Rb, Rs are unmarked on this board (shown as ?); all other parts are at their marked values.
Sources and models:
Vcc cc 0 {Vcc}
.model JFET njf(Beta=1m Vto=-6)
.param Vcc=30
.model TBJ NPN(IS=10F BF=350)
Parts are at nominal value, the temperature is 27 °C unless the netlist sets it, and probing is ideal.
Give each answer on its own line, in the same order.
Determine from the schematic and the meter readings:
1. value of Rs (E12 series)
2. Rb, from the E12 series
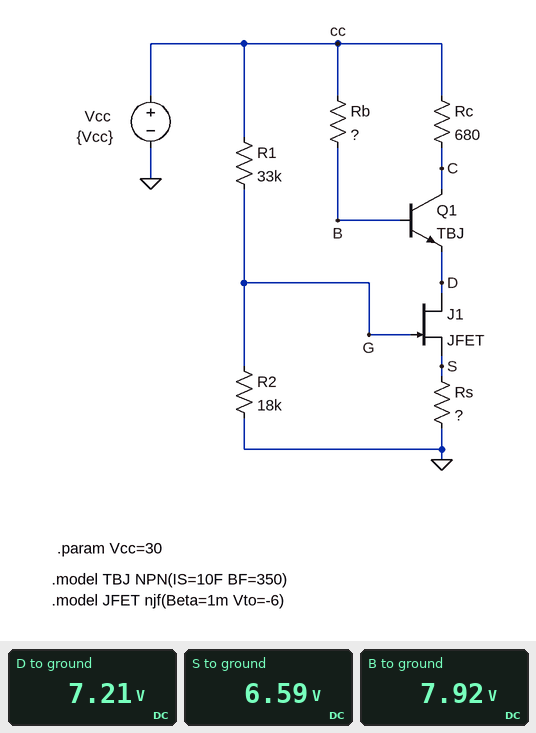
820 Ω
1 MΩ
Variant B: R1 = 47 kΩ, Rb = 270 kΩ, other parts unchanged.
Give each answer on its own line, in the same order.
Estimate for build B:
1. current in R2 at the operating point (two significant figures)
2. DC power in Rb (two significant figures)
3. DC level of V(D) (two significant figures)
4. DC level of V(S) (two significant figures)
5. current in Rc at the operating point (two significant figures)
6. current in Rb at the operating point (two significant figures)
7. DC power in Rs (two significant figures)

460 µA
370 µW
19 V
11 V
13 mA
37 µA
140 mW
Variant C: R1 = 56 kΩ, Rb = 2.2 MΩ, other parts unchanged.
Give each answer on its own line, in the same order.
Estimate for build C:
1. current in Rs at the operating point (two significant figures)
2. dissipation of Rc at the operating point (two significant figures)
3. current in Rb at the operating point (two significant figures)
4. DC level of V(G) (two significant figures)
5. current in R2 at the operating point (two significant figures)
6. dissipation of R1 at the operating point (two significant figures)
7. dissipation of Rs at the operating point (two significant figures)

4.3 mA
11 mW
12 µA
4.1 V
230 µA
12 mW
15 mW
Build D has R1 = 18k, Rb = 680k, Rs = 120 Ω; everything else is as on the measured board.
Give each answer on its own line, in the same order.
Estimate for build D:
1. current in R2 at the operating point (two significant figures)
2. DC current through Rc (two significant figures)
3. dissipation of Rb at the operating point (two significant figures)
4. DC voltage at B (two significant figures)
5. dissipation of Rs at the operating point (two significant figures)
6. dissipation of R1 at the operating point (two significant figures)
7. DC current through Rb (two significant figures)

140 µA
14 mA
1.0 mW
3.6 V
27 mW
42 mW
39 µA
